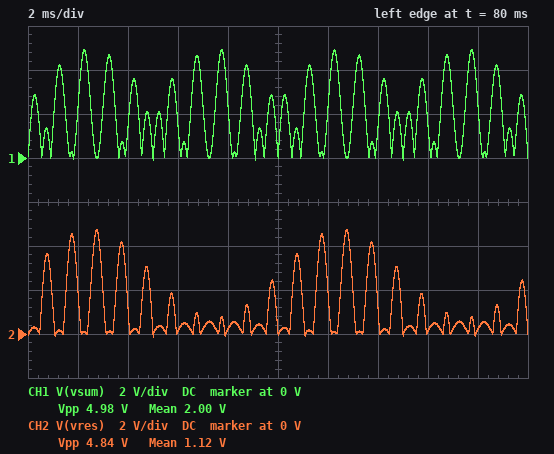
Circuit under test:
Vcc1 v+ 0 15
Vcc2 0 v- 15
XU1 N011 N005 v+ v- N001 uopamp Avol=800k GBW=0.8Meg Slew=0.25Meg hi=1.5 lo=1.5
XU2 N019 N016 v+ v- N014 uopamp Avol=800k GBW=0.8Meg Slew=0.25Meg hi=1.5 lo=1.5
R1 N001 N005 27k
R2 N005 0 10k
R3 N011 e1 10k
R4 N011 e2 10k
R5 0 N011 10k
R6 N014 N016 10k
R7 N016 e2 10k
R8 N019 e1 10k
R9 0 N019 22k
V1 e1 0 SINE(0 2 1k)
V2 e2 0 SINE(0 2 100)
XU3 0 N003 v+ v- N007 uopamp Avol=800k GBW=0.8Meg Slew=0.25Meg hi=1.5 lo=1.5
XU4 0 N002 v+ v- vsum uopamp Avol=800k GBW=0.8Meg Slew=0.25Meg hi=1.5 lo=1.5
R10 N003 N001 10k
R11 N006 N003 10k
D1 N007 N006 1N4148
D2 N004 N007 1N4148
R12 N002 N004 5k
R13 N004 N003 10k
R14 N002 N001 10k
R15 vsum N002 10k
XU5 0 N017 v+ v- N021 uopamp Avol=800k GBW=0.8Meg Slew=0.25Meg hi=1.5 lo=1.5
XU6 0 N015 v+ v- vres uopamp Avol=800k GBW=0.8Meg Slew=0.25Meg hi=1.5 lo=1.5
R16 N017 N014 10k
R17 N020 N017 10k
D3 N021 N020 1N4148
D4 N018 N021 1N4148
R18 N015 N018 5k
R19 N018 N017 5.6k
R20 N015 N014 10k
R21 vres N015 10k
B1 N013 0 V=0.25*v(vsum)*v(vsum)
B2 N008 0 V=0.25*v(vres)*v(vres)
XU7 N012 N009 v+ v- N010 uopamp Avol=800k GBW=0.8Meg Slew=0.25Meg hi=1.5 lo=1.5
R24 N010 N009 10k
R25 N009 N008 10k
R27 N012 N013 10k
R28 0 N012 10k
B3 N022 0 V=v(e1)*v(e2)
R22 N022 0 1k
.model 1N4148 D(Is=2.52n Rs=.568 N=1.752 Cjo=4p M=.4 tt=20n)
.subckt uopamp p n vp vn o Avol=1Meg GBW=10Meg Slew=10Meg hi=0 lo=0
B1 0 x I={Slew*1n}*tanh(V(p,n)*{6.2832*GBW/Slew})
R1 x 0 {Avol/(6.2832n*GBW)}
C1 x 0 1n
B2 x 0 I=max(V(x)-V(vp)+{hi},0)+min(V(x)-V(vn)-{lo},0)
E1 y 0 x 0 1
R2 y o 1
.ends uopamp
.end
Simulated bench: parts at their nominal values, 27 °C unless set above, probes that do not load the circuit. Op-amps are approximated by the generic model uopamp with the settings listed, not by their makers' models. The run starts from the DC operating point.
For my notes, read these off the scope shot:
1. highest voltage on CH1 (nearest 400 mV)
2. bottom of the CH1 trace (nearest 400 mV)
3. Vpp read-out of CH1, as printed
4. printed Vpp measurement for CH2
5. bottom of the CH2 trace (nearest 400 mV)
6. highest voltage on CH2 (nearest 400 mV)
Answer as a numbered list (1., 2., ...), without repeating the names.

1. 4.8 V
2. 0 V
3. 4.98 V
4. 4.84 V
5. 0 V
6. 4.8 V
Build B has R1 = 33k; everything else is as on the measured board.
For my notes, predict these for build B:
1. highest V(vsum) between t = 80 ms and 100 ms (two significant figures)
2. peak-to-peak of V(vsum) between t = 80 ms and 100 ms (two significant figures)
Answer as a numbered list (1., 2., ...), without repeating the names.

1. 5.7 V
2. 5.8 V
